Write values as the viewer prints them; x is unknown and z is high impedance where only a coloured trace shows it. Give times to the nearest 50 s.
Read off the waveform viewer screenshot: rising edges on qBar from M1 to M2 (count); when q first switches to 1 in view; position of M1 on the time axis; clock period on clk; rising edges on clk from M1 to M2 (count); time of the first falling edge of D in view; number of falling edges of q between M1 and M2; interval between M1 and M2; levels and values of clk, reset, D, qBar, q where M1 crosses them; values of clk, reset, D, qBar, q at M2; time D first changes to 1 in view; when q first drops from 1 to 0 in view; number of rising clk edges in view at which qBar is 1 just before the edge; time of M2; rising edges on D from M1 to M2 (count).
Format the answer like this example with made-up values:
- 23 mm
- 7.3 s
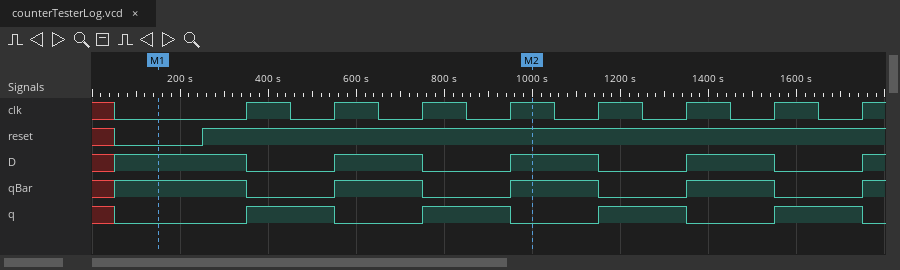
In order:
- 2
- 350 s
- 150 s
- 200 s
- 4
- 350 s
- 2
- 850 s
- clk=0, reset=0, D=1, qBar=1, q=0
- clk=1, reset=1, D=1, qBar=1, q=0
- 50 s
- 550 s
- 4
- 1000 s
- 2
